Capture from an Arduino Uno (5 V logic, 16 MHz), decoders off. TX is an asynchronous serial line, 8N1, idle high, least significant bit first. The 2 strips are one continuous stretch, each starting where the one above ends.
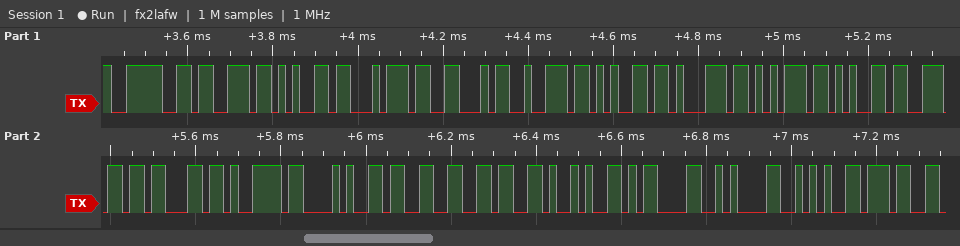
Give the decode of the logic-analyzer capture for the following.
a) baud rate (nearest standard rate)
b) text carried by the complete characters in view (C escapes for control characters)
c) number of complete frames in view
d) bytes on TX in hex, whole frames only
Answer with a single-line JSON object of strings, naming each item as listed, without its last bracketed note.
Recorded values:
{"baud rate": "57600 baud", "text carried by the complete characters in view": "\">setFrequency(36)\\r\\n*7\"", "number of complete frames in view": "21", "bytes on TX in hex, whole frames only": "3E 73 65 74 46 72 65 71 75 65 6E 63 79 28 33 36 29 0D 0A 2A 37"}
